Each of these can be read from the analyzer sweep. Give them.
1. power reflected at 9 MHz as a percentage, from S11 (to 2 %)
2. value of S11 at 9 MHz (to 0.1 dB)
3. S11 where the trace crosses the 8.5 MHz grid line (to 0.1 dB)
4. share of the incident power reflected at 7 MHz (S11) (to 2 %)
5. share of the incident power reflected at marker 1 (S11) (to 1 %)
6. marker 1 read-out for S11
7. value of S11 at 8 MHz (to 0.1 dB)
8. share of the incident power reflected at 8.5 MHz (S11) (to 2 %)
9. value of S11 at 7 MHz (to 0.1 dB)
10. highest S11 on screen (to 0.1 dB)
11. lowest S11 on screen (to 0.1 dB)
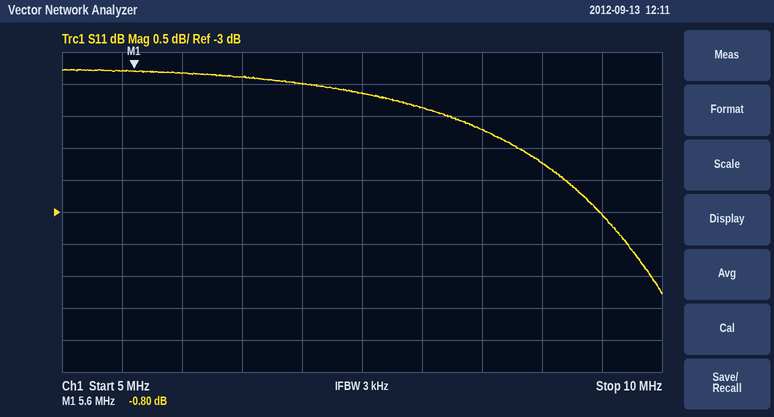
60 %
-2.2 dB
-1.7 dB
80 %
83 %
-0.80 dB
-1.4 dB
68 %
-1.0 dB
-0.8 dB
-4.3 dB
